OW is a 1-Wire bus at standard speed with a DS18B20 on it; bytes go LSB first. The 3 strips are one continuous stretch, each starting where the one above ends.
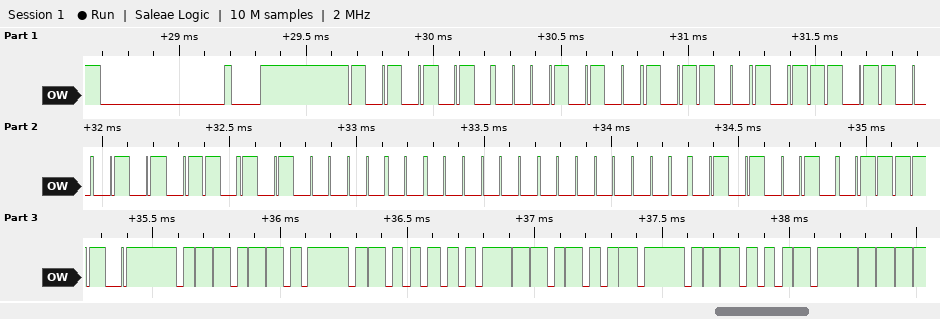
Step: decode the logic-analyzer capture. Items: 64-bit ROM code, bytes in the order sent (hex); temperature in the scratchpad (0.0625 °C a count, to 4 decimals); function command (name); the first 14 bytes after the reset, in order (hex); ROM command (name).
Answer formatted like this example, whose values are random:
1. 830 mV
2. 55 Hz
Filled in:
1. 28 4D 37 6A 05 00 00 4A
2. 35.3750 °C
3. Read Scratchpad
4. 55 28 4D 37 6A 05 00 00 4A BE 36 02 4B 46
5. Match ROM
